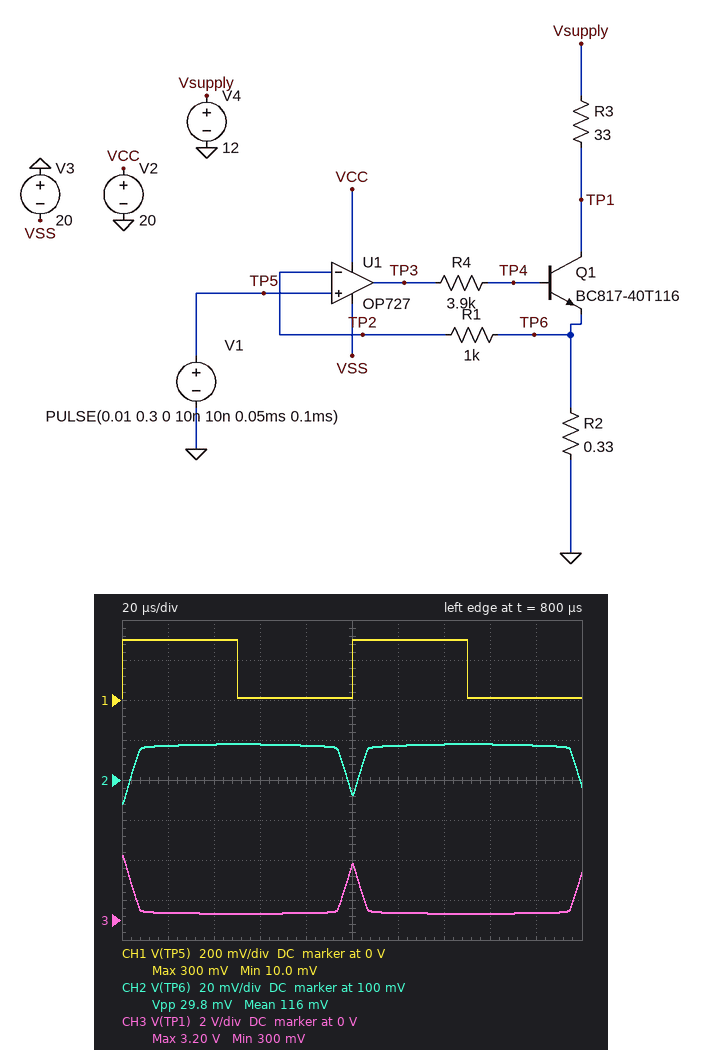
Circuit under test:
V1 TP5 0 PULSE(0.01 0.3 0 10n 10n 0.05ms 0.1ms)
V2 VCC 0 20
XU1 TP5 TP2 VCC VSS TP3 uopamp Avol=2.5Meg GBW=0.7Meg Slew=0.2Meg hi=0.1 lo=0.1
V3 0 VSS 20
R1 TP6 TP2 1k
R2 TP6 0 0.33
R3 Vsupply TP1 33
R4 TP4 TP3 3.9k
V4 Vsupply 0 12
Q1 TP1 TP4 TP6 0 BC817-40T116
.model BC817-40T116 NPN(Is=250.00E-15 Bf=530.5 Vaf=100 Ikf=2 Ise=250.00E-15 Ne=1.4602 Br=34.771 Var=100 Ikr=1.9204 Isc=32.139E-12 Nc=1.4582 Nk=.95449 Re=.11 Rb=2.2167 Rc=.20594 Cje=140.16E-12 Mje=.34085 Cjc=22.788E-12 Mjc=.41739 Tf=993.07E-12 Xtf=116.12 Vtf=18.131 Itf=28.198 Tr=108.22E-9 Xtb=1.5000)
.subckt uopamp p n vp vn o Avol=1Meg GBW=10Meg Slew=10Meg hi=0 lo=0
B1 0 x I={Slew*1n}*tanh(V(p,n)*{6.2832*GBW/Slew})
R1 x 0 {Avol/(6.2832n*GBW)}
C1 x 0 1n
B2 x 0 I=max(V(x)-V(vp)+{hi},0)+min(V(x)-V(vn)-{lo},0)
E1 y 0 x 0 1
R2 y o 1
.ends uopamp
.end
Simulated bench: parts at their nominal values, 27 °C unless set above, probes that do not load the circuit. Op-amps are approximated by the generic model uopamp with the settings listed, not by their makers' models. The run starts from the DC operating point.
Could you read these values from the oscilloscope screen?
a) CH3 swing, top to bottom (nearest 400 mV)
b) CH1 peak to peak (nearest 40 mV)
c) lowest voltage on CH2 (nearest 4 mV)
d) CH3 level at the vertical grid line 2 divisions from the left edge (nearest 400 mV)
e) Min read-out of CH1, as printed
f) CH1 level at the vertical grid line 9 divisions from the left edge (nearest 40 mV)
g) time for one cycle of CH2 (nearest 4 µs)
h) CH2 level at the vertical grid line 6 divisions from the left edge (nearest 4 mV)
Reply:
2.8 V
280 mV
88 mV
400 mV
10.0 mV
0 V
100 µs
116 mV
